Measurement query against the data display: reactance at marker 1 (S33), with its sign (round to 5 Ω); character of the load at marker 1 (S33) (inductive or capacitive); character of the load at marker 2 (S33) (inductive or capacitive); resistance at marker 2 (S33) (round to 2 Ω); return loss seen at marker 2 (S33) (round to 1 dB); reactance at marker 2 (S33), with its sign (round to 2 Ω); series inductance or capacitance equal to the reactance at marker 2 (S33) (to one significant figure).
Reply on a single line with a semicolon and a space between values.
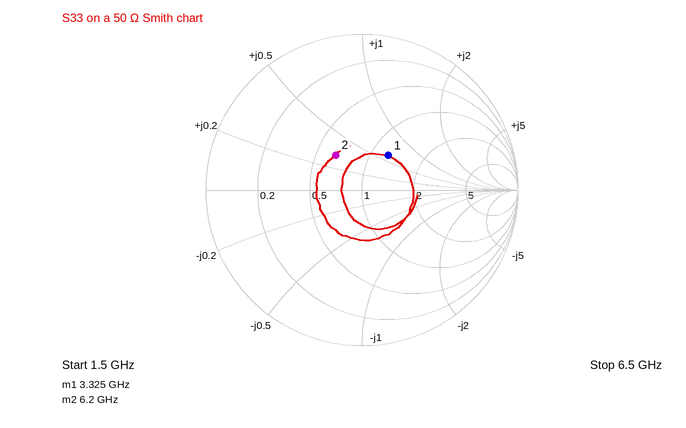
+30 Ω; inductive; inductive; 32 Ω; 11 dB; +16 Ω; 400 pH
